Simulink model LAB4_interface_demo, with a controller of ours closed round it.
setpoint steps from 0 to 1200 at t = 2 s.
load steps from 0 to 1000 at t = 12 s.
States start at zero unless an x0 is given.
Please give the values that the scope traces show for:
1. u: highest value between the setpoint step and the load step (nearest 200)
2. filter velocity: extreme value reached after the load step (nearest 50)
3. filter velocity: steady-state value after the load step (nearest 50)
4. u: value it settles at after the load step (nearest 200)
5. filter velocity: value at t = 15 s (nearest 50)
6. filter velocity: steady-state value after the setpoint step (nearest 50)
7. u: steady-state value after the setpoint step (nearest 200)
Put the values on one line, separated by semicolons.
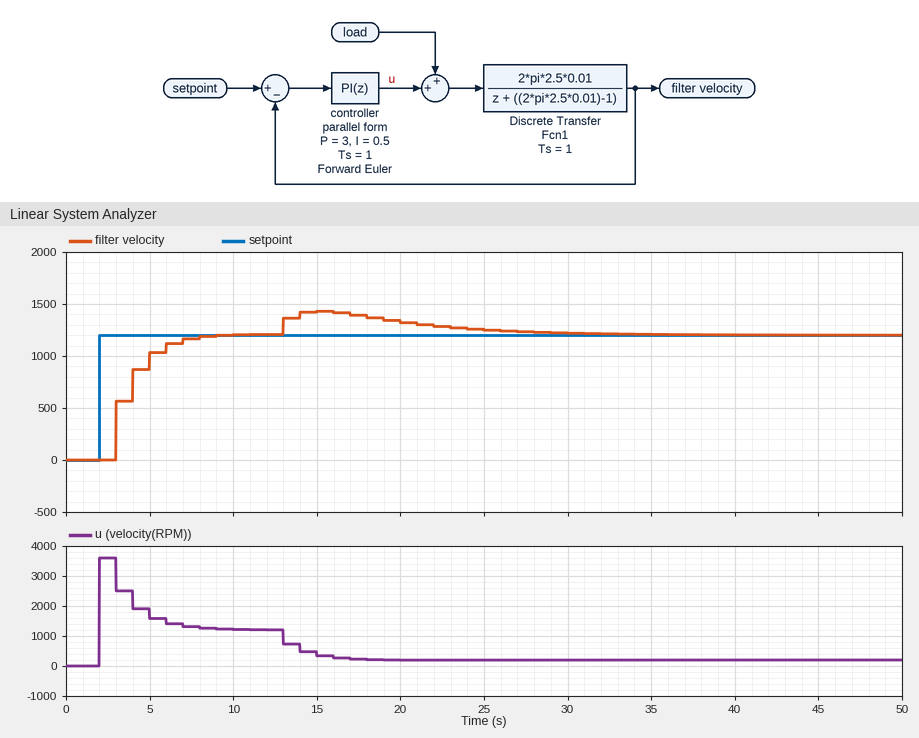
3600; 1450; 1200; 200; 1450; 1200; 1200
